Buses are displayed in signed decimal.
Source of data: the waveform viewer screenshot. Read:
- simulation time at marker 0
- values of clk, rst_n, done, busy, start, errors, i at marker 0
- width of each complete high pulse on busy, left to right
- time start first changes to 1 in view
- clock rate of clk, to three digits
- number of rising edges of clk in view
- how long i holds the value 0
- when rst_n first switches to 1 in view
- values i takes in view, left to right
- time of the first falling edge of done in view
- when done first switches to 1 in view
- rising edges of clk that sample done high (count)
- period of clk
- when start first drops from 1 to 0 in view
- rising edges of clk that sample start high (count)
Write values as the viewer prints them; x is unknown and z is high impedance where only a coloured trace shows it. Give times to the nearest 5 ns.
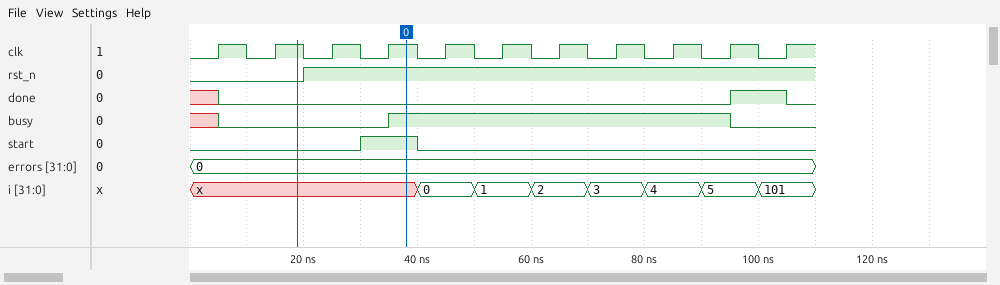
40 ns
clk=1, rst_n=1, done=0, busy=1, start=1, errors=0, i=x
60 ns
30 ns
100 MHz
11
10 ns
20 ns
x, 0, 1, 2, 3, 4, 5, 101
105 ns
95 ns
1
10 ns
40 ns
1
